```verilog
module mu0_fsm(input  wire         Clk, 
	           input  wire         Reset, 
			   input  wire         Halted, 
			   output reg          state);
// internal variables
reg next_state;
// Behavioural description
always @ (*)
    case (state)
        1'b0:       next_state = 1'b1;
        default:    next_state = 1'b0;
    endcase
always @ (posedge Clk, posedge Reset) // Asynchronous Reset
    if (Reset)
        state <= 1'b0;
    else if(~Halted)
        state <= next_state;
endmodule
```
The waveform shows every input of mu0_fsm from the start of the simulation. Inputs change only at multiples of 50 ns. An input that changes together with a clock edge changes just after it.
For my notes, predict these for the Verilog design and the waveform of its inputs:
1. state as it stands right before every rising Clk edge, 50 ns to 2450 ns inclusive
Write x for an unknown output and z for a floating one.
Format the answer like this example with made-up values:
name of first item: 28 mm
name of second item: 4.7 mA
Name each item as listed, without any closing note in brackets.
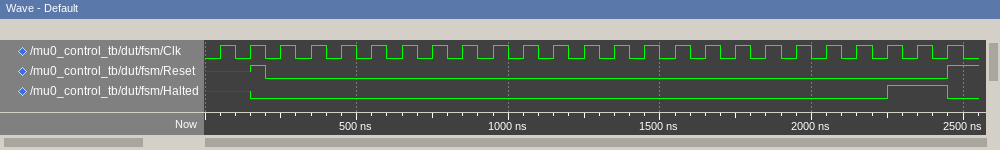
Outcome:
state as it stands right before every rising Clk edge, 50 ns to 2450 ns inclusive: x x 0 1 0 1 0 1 0 1 0 1 0 1 0 1 0 1 0 1 0 1 0 1 1
